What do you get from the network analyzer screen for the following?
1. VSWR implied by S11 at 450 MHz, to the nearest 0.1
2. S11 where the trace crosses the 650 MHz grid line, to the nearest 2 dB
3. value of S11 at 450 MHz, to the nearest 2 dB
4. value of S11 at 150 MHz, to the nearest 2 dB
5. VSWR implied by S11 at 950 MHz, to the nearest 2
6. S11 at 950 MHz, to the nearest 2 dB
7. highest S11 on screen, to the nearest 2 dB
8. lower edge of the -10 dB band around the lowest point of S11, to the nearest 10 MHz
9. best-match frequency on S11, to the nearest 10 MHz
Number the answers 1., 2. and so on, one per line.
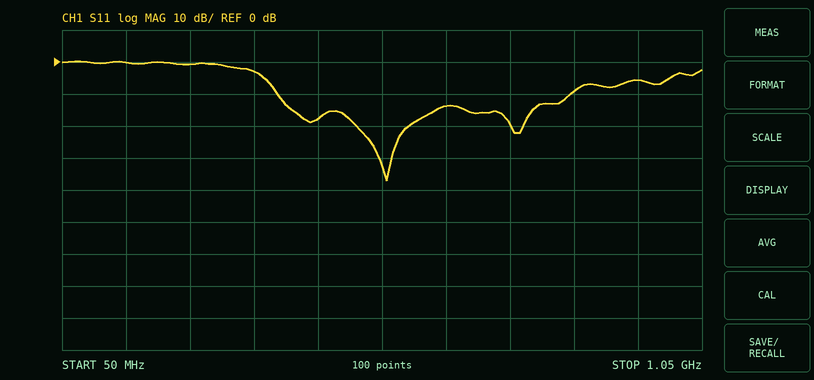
1. 1.3
2. -14 dB
3. -18 dB
4. 0 dB
5. 4
6. -6 dB
7. 0 dB
8. 390 MHz
9. 560 MHz
